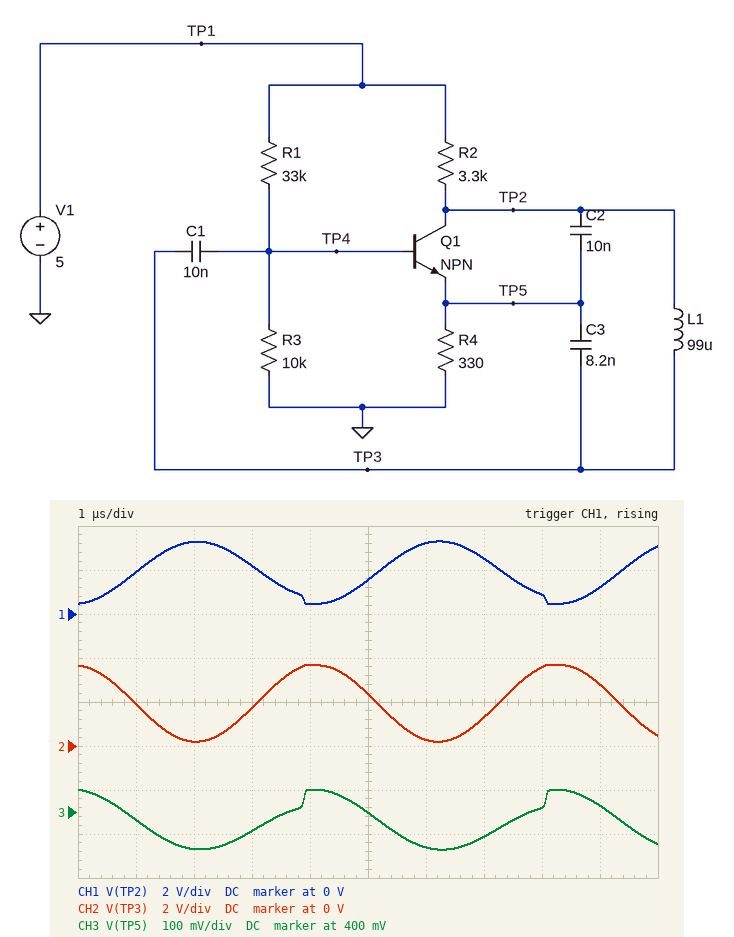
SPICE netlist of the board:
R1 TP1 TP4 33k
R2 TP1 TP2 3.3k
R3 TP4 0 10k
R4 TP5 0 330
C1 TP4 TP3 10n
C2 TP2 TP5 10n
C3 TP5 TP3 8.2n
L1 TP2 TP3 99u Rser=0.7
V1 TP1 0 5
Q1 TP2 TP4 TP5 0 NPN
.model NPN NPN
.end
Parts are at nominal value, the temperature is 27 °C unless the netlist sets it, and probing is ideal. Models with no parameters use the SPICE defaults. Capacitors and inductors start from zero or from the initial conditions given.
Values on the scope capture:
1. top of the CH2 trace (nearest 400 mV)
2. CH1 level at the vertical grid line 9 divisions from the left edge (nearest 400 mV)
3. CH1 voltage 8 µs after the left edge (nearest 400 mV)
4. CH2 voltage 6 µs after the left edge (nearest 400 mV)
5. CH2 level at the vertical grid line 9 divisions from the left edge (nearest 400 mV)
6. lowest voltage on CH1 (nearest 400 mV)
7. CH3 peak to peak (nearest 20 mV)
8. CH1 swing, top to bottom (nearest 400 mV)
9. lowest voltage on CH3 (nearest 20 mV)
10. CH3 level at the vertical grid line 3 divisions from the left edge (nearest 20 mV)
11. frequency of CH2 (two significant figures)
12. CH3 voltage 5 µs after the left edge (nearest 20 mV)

3.6 V
1.2 V
800 mV
400 mV
2.8 V
400 mV
140 mV
2.8 V
320 mV
360 mV
240 kHz
400 mV
